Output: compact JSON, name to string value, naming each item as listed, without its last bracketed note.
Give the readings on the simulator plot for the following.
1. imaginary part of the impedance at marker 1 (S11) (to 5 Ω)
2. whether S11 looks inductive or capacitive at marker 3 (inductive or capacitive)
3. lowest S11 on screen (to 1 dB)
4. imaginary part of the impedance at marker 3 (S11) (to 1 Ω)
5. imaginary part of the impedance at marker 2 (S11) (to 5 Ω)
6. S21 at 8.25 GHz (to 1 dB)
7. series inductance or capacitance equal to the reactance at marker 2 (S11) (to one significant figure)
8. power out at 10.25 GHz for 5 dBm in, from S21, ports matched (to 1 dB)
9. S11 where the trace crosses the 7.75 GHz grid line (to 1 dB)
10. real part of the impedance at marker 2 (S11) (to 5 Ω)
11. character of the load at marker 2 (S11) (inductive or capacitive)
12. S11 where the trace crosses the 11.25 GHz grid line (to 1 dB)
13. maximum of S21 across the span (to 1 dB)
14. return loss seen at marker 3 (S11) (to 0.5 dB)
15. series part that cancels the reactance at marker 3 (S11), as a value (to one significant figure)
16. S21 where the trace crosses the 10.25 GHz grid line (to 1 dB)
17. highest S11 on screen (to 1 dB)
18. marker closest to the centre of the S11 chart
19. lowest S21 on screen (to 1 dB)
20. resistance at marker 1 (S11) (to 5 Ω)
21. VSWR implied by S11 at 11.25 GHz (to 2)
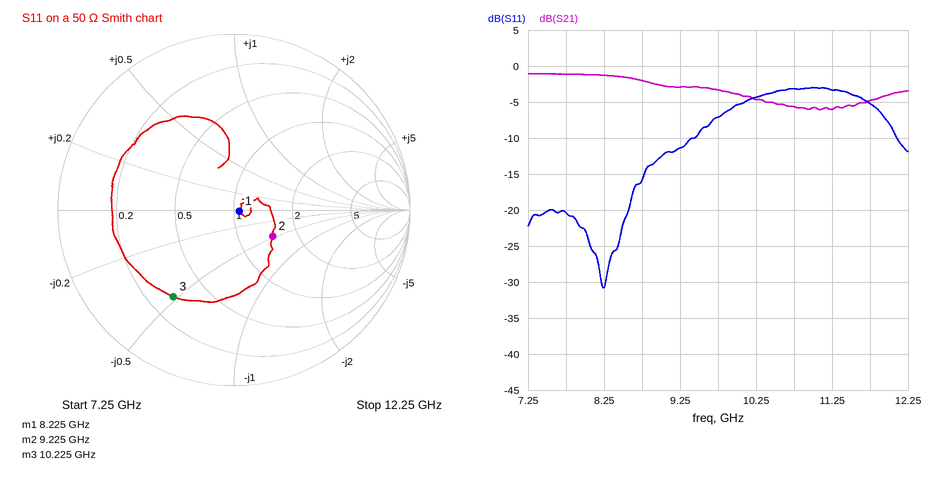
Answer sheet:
{"imaginary part of the impedance at marker 1 (S11)": "0 Ω", "whether S11 looks inductive or capacitive at marker 3": "capacitive", "lowest S11 on screen": "-31 dB", "imaginary part of the impedance at marker 3 (S11)": "-24 Ω", "imaginary part of the impedance at marker 2 (S11)": "-25 Ω", "S21 at 8.25 GHz": "-1 dB", "series inductance or capacitance equal to the reactance at marker 2 (S11)": "700 fF", "power out at 10.25 GHz for 5 dBm in, from S21, ports matched": "0 dBm", "S11 where the trace crosses the 7.75 GHz grid line": "-20 dB", "real part of the impedance at marker 2 (S11)": "75 Ω", "character of the load at marker 2 (S11)": "capacitive", "S11 where the trace crosses the 11.25 GHz grid line": "-3 dB", "maximum of S21 across the span": "-1 dB", "return loss seen at marker 3 (S11)": "4.5 dB", "series part that cancels the reactance at marker 3 (S11), as a value": "400 pH", "S21 where the trace crosses the 10.25 GHz grid line": "-5 dB", "highest S11 on screen": "-3 dB", "marker closest to the centre of the S11 chart": "marker 1", "lowest S21 on screen": "-6 dB", "resistance at marker 1 (S11)": "55 Ω", "VSWR implied by S11 at 11.25 GHz": "6"}
